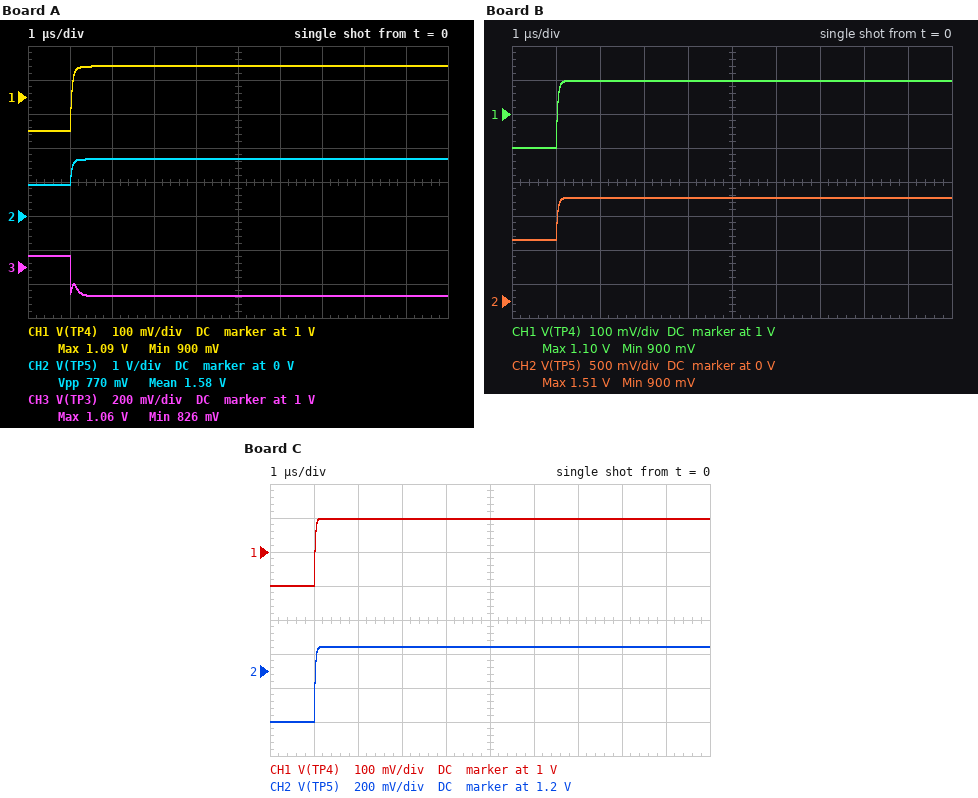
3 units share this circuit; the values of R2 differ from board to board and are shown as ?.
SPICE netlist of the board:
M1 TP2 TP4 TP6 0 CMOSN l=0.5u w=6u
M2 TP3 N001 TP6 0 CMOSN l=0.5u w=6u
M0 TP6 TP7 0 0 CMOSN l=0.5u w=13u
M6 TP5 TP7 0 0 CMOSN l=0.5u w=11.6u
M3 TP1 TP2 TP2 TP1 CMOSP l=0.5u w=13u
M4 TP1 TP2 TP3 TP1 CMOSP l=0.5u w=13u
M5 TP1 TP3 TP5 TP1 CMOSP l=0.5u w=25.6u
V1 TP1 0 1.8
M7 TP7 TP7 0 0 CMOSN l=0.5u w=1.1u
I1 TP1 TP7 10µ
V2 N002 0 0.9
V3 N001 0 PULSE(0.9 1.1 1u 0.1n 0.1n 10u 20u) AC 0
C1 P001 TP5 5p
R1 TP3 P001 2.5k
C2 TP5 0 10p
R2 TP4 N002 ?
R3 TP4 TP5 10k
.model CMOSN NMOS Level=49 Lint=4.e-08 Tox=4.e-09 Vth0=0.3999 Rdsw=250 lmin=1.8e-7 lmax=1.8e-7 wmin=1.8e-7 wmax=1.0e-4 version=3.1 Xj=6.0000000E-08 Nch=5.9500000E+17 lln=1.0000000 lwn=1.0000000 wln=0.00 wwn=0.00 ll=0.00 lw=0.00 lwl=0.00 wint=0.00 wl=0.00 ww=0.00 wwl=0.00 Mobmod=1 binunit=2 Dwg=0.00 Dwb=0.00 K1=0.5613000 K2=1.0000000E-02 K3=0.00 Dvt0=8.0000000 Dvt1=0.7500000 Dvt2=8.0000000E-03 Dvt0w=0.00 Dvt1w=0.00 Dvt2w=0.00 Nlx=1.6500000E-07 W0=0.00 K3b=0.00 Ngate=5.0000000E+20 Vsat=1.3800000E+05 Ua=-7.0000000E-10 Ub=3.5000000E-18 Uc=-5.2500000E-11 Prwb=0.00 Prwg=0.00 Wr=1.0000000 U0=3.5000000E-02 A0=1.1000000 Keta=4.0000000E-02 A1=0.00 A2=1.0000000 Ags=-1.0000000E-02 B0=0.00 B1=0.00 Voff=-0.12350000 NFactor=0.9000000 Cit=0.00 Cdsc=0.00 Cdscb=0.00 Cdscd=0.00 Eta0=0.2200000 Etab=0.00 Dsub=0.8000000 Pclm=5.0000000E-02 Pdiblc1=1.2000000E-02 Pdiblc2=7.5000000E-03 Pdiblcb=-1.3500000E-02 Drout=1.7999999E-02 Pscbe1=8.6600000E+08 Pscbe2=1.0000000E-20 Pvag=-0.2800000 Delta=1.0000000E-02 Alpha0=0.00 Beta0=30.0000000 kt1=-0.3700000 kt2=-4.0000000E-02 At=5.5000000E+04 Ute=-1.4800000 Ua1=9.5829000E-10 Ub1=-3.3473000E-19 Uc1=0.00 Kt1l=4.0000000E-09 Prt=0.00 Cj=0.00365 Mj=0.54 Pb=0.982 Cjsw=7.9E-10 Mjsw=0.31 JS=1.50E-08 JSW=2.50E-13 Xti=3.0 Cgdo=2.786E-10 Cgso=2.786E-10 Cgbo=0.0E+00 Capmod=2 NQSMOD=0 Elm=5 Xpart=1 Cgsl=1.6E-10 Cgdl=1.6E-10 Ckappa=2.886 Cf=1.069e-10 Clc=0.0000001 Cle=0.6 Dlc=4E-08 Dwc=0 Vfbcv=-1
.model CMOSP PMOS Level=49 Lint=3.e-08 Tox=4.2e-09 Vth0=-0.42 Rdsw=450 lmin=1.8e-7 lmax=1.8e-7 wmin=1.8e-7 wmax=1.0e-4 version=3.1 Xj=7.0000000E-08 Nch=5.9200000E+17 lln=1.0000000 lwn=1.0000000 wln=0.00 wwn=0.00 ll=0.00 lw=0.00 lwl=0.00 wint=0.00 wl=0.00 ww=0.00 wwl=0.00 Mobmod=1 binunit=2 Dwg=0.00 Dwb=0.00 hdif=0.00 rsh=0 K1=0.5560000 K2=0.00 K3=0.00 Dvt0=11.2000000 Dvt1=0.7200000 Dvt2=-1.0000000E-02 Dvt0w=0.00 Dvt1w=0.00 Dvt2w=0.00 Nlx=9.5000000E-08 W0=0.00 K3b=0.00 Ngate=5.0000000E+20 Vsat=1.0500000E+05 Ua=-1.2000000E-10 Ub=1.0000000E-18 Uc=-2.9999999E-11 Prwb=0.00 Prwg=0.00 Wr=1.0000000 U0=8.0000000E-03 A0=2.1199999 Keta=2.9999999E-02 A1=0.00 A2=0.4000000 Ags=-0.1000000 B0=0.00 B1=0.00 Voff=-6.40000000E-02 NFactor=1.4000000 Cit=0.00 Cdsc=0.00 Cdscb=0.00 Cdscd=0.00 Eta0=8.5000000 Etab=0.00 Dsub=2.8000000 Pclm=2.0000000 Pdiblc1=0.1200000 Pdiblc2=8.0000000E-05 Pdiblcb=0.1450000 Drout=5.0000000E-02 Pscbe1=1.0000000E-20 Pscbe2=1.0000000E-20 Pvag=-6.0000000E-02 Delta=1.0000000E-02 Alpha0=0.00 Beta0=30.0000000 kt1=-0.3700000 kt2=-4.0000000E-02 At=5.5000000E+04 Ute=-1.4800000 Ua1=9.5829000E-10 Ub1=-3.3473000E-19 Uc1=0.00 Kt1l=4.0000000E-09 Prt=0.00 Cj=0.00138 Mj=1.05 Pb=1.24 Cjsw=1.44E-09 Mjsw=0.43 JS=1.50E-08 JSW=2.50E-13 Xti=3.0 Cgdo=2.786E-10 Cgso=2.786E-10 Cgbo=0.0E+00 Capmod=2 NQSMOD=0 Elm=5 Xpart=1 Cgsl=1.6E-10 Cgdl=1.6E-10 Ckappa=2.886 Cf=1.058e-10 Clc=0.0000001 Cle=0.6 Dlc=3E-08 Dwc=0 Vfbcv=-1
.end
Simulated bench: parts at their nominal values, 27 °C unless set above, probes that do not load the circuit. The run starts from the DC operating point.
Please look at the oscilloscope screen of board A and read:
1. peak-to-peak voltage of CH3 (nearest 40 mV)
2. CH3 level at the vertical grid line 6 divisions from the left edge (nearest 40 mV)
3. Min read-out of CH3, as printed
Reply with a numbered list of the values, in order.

1. 240 mV
2. 840 mV
3. 826 mV
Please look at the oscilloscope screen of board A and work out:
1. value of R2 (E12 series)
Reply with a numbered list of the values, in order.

1. 3.3 kΩ
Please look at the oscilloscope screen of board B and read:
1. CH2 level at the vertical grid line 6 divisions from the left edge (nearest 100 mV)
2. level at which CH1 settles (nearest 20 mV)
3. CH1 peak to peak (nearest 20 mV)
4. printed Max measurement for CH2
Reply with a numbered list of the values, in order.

1. 1.5 V
2. 1.10 V
3. 200 mV
4. 1.51 V
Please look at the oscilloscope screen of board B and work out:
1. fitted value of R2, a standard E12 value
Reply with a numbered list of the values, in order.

1. 4.7 kΩ
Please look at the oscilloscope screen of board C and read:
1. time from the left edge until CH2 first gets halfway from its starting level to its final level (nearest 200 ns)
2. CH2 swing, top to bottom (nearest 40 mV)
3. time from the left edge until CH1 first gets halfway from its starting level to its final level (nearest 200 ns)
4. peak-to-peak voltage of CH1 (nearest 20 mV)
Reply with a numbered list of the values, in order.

1. 1.0 µs
2. 440 mV
3. 1.0 µs
4. 200 mV
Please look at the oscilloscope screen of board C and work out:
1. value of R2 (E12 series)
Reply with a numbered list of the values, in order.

1. 8.2 kΩ
